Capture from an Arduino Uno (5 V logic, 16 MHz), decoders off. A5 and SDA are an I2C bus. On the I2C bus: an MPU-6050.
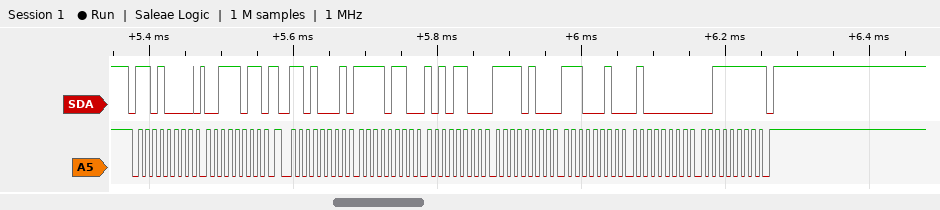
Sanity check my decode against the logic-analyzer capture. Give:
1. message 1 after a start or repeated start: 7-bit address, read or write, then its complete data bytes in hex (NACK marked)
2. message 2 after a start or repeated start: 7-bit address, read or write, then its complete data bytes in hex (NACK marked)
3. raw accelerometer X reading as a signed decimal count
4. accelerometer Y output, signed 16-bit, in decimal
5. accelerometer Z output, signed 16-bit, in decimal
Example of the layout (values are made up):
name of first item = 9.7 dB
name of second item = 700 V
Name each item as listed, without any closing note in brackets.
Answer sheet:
message 1 after a start or repeated start: 7-bit address, read or write, then its complete data bytes in hex = 0x68 write: 3B
message 2 after a start or repeated start: 7-bit address, read or write, then its complete data bytes in hex = 0x68 read: F6 AC F4 E2 40 3F NACK
raw accelerometer X reading as a signed decimal count = -2388
accelerometer Y output, signed 16-bit, in decimal = -2846
accelerometer Z output, signed 16-bit, in decimal = 16447
